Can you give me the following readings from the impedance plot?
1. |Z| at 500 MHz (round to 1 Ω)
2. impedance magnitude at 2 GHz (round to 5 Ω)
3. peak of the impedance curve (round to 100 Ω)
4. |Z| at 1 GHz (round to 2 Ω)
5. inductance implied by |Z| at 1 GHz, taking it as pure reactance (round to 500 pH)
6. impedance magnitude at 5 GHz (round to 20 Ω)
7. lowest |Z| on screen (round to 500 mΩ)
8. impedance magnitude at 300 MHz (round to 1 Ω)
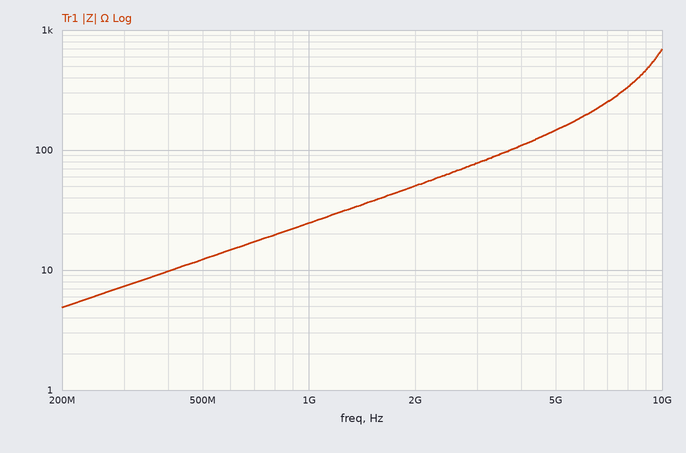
12 Ω
50 Ω
700 Ω
24 Ω
4.0 nH
140 Ω
5.0 Ω
7 Ω
